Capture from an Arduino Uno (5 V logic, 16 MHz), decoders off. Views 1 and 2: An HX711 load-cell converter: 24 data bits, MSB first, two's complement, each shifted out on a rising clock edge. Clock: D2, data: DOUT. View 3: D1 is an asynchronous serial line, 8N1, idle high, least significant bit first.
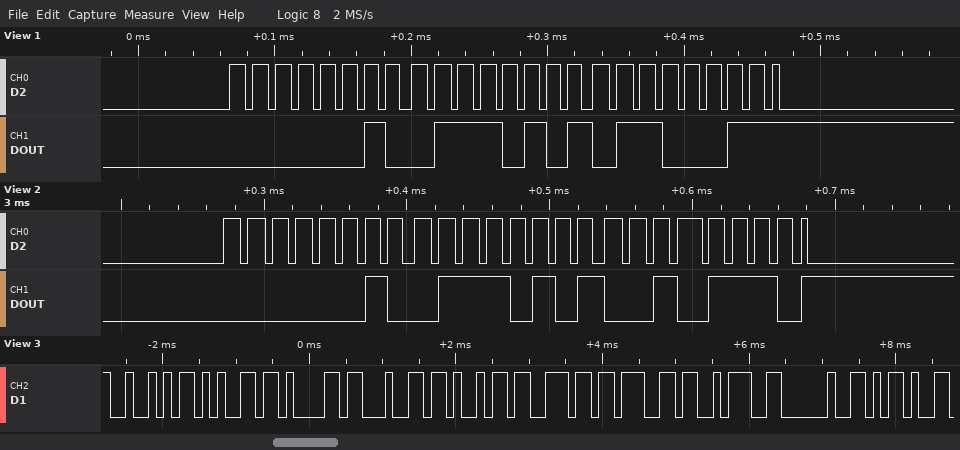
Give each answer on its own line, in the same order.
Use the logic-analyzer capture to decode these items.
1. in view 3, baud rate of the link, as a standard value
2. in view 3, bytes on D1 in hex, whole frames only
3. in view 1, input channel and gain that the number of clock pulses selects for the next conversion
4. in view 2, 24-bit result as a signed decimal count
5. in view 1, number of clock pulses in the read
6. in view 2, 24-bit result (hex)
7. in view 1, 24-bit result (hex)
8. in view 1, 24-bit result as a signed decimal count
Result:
9600 baud
52 65 61 64 69 6E 67 3A 20 2D
channel A, gain 128
161070
25
0x02752E
0x027563
161123
